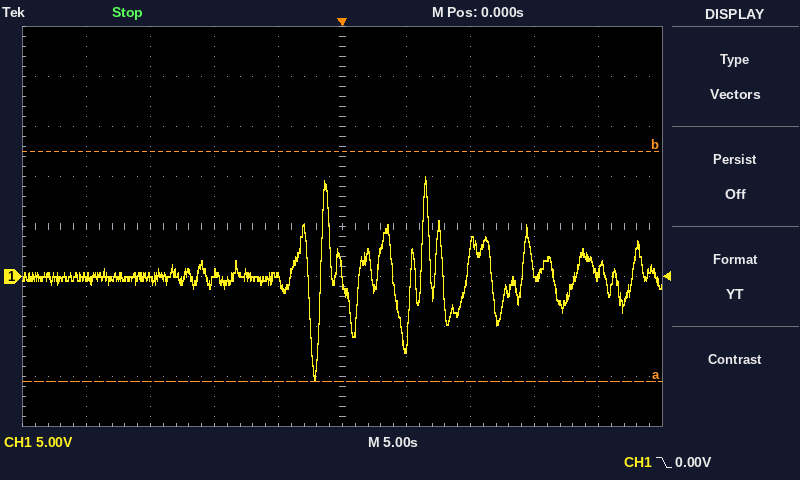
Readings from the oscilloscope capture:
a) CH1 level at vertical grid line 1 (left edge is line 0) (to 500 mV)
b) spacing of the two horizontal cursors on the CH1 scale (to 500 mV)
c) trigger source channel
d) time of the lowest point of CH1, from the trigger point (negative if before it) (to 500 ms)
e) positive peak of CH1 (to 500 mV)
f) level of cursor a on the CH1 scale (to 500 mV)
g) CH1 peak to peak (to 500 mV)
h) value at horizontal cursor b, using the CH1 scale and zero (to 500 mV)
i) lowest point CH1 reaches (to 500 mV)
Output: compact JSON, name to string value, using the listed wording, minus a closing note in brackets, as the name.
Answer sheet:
{"CH1 level at vertical grid line 1 (left edge is line 0)": "0.0 V", "spacing of the two horizontal cursors on the CH1 scale": "23.0 V", "trigger source channel": "CH1", "time of the lowest point of CH1, from the trigger point (negative if before it)": "-2.0 s", "positive peak of CH1": "10.0 V", "level of cursor a on the CH1 scale": "-10.5 V", "CH1 peak to peak": "20.5 V", "value at horizontal cursor b, using the CH1 scale and zero": "12.5 V", "lowest point CH1 reaches": "-10.5 V"}
